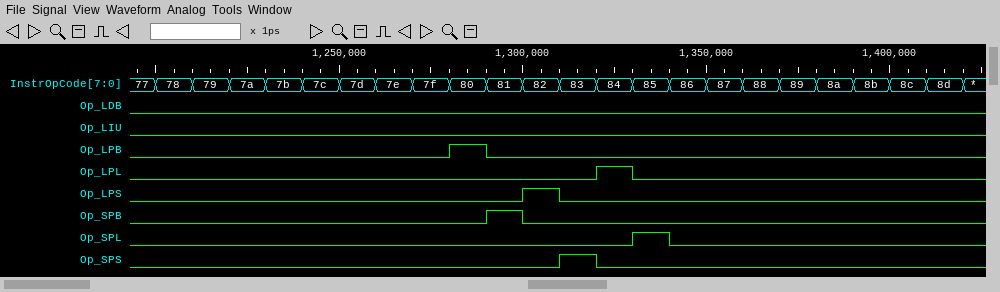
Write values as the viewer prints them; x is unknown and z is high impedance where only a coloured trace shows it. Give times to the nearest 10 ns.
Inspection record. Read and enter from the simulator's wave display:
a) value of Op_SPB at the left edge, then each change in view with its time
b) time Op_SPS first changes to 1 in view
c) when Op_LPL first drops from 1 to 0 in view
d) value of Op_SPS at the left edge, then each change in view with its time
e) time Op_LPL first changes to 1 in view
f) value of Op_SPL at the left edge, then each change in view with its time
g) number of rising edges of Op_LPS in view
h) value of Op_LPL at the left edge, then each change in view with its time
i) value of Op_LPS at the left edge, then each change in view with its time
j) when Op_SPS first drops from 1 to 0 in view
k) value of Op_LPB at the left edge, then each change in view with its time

0, 1 at 1290 ns, 0 at 1300 ns
1310 ns
1330 ns
0, 1 at 1310 ns, 0 at 1320 ns
1320 ns
0, 1 at 1330 ns, 0 at 1340 ns
1
0, 1 at 1320 ns, 0 at 1330 ns
0, 1 at 1300 ns, 0 at 1310 ns
1320 ns
0, 1 at 1280 ns, 0 at 1290 ns
